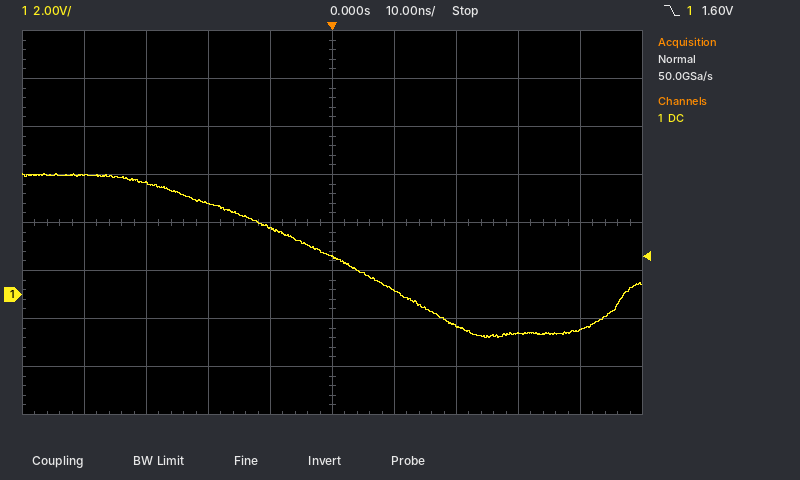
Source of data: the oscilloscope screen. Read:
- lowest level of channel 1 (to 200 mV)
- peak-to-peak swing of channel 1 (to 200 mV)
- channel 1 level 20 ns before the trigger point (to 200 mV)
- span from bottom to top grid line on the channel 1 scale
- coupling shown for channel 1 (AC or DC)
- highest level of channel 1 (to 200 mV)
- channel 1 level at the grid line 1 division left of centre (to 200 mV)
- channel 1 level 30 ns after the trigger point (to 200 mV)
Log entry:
-1.8 V
6.8 V
3.8 V
16 V
DC
5.0 V
2.8 V
-1.6 V
